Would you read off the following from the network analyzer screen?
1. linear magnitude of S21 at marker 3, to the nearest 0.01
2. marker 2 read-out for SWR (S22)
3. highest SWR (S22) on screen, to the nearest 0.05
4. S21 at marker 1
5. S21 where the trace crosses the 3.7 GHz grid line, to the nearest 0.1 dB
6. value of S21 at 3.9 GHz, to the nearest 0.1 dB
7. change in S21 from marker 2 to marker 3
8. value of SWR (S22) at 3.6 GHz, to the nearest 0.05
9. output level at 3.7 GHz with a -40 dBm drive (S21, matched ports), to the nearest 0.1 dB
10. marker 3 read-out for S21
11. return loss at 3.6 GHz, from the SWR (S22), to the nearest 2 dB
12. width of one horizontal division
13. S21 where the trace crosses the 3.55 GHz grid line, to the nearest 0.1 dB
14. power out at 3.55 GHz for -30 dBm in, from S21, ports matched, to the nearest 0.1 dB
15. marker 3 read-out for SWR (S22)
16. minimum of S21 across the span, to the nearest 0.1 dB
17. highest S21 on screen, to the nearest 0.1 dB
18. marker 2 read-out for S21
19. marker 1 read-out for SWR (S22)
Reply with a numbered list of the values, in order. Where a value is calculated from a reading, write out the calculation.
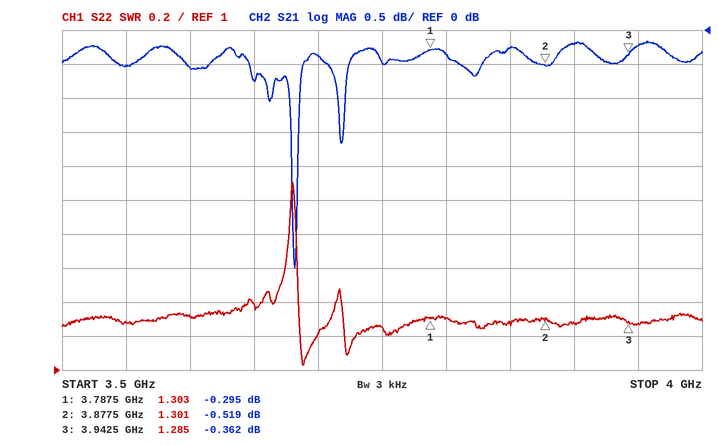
1. 10^(-0.362/20) ≈ 0.96
2. 1.301
3. 2.10
4. -0.295 dB
5. -0.4 dB
6. -0.2 dB
7. -0.362 − (-0.519) = 0.157 dB
8. 1.30
9. -40 dBm + (-0.4 dB) = -40.4 dBm
10. -0.362 dB
11. −20 log10((1.3 − 1)/(1.3 + 1)) ≈ 18 dB
12. 50 MHz
13. -0.5 dB
14. -30 dBm + (-0.5 dB) = -30.5 dBm
15. 1.285
16. -3.5 dB
17. -0.2 dB
18. -0.519 dB
19. 1.303
